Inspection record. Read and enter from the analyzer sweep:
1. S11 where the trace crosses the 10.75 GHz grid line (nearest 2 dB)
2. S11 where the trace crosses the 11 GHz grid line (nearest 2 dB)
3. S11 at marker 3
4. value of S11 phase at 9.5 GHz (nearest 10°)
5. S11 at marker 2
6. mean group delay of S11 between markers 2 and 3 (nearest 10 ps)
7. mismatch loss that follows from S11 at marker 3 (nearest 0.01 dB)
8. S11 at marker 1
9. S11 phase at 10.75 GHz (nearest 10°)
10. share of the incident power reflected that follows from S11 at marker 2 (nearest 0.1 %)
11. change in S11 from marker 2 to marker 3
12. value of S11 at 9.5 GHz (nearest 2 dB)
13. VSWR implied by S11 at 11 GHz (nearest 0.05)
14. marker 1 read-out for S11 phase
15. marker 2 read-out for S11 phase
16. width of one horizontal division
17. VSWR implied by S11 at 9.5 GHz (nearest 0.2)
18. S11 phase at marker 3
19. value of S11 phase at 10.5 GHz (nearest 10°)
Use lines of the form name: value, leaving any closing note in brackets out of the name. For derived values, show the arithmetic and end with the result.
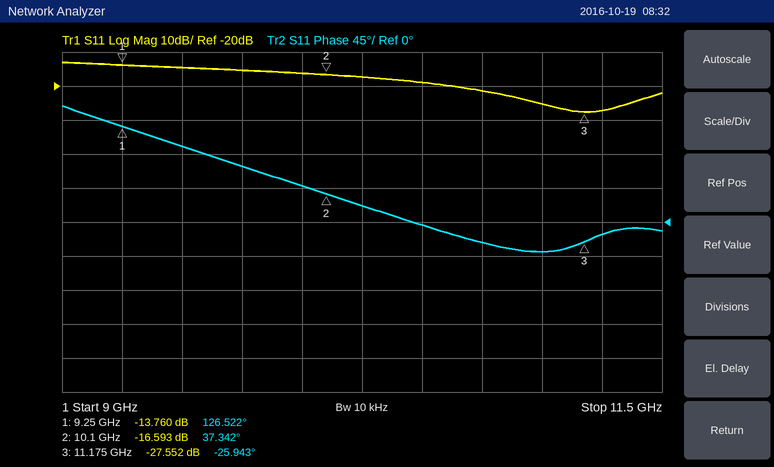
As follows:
S11 where the trace crosses the 10.75 GHz grid line: -22 dB
S11 where the trace crosses the 11 GHz grid line: -26 dB
S11 at marker 3: -27.552 dB
value of S11 phase at 9.5 GHz: 100°
S11 at marker 2: -16.593 dB
mean group delay of S11 between markers 2 and 3: −(-25.943° − (37.342°))/(360° × 1.075 GHz) ≈ 164 ps, so 160 ps to the nearest 10 ps
mismatch loss that follows from S11 at marker 3: −10 log10(1 − 10^(-27.552/10)) ≈ 0.01 dB
S11 at marker 1: -13.760 dB
S11 phase at 10.75 GHz: -30°
share of the incident power reflected that follows from S11 at marker 2: 10^(-16.593/10) ≈ 2.2 %
change in S11 from marker 2 to marker 3: -27.552 − (-16.593) = -10.959 dB
value of S11 at 9.5 GHz: -14 dB
VSWR implied by S11 at 11 GHz: |Γ| = 10^(-26/20) = 0.0501; VSWR = (1 + 0.0501)/(1 − 0.0501) ≈ 1.11, so 1.10 to the nearest 0.05
marker 1 read-out for S11 phase: 126.522°
marker 2 read-out for S11 phase: 37.342°
width of one horizontal division: 250 MHz
VSWR implied by S11 at 9.5 GHz: |Γ| = 10^(-14/20) = 0.1995; VSWR = (1 + 0.1995)/(1 − 0.1995) ≈ 1.50, so 1.4 to the nearest 0.2
S11 phase at marker 3: -25.943°
value of S11 phase at 10.5 GHz: 0°
